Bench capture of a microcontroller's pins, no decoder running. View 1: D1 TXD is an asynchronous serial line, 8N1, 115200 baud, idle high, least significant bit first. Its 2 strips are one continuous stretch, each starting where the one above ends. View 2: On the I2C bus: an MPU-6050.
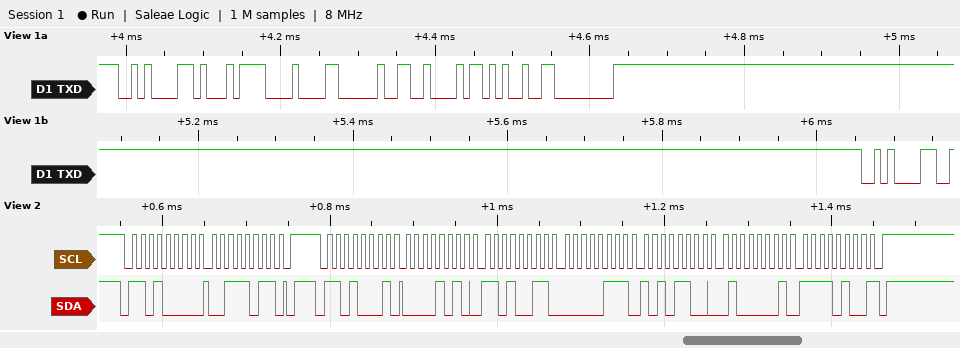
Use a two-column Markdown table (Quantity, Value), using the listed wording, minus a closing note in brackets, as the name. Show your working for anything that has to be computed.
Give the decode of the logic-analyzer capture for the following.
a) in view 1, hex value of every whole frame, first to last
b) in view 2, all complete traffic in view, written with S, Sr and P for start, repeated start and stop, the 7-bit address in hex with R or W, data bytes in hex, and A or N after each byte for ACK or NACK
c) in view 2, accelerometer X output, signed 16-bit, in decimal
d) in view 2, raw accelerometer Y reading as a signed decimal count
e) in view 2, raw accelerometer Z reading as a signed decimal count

| Quantity | Value |
|---|---|
| in view 1, hex value of every whole frame, first to last | 0A D1 08 20 42 25 00 0A |
| in view 2, all complete traffic in view, written with S, Sr and P for start, repeated start and stop, the 7-bit address in hex with R or W, data bytes in hex, and A or N after each byte for ACK or NACK | S 68W A 3B A P S 68R A 0A A D3 A 07 A AC A 41 A F4 N P |
| in view 2, accelerometer X output, signed 16-bit, in decimal | 0x0AD3 = 2771 |
| in view 2, raw accelerometer Y reading as a signed decimal count | 0x07AC = 1964 |
| in view 2, raw accelerometer Z reading as a signed decimal count | 0x41F4 = 16884 |
